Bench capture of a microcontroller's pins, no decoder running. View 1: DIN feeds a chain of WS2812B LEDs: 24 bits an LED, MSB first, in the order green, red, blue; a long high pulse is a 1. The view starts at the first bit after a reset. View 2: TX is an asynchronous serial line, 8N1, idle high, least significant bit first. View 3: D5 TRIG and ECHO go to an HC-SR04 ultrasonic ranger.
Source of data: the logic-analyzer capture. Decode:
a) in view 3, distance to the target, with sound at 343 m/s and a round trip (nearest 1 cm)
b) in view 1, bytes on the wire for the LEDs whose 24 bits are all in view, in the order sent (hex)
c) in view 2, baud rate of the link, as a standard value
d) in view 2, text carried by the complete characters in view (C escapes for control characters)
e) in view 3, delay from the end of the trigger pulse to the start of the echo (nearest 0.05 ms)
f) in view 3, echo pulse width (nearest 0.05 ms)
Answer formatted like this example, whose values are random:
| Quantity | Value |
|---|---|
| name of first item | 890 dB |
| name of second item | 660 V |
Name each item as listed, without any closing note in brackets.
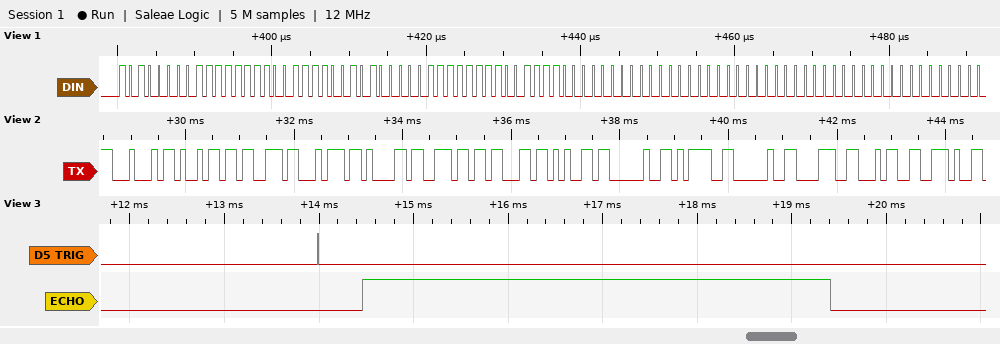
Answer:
| Quantity | Value |
|---|---|
| in view 3, distance to the target, with sound at 343 m/s and a round trip | 85 cm |
| in view 1, bytes on the wire for the LEDs whose 24 bits are all in view, in the order sent | A0 FF 3C A0 FF 3C 00 00 00 |
| in view 2, baud rate of the link, as a standard value | 9600 baud |
| in view 2, text carried by the complete characters in view | "Distance = 84." |
| in view 3, delay from the end of the trigger pulse to the start of the echo | 0.45 ms |
| in view 3, echo pulse width | 4.95 ms |
